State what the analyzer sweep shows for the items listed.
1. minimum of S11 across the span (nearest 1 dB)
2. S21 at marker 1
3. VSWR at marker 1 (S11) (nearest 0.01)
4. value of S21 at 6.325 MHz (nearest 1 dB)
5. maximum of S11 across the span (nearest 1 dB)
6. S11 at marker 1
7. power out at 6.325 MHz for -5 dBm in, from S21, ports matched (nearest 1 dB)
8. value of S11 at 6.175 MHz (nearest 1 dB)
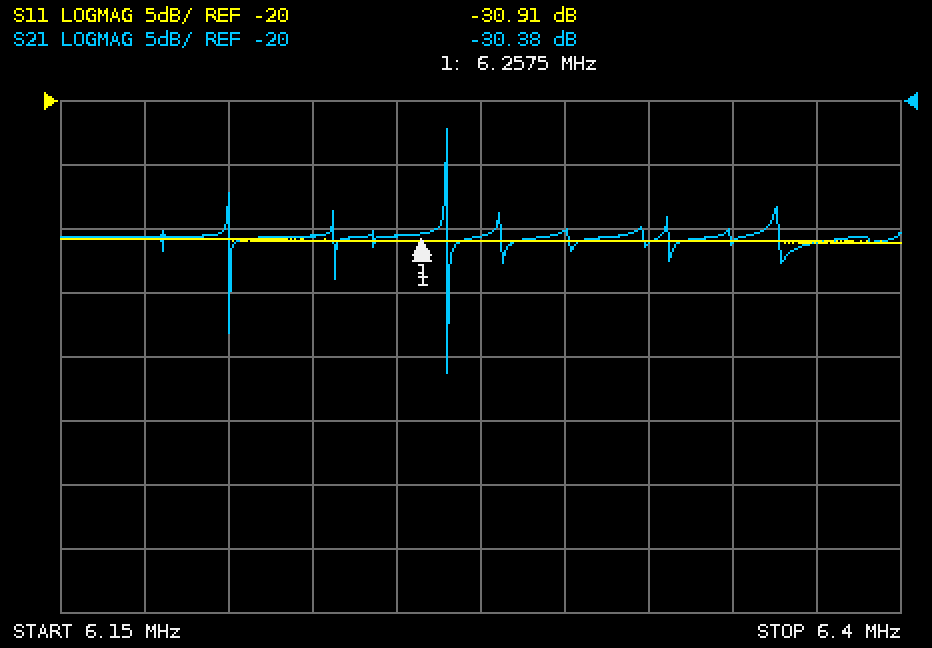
-31 dB
-30.38 dB
1.06
-31 dB
-31 dB
-30.91 dB
-36 dBm
-31 dB
